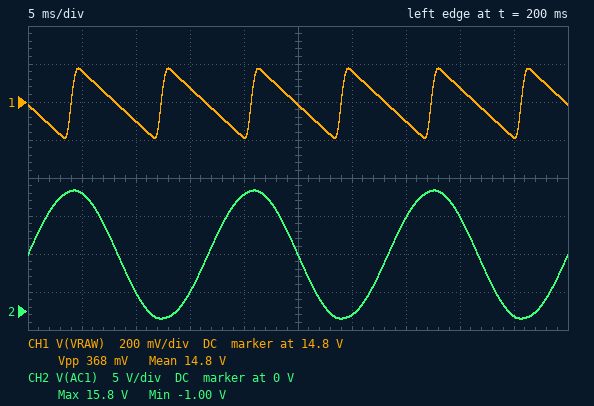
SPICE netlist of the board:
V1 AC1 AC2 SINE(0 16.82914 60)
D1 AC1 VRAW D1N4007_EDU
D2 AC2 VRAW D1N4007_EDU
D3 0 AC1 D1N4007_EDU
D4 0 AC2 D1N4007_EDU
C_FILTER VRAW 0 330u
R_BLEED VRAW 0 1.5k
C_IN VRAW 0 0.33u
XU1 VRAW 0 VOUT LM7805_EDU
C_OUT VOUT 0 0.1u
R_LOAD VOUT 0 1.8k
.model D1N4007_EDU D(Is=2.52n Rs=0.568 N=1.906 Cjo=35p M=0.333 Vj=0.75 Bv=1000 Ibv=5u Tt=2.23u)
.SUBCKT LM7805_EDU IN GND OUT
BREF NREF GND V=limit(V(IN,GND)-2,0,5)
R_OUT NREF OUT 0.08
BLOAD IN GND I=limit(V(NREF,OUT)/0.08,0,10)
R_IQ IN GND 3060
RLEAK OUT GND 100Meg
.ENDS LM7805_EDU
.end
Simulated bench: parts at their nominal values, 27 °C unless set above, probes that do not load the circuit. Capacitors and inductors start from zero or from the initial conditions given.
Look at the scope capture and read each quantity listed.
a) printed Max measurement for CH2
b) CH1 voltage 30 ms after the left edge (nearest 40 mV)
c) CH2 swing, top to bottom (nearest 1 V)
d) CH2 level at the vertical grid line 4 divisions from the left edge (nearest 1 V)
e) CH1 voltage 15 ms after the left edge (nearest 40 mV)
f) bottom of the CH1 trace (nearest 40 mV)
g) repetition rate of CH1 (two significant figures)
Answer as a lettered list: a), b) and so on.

a) 15.8 V
b) 14.96 V
c) 17 V
d) 15 V
e) 14.88 V
f) 14.60 V
g) 120 Hz
